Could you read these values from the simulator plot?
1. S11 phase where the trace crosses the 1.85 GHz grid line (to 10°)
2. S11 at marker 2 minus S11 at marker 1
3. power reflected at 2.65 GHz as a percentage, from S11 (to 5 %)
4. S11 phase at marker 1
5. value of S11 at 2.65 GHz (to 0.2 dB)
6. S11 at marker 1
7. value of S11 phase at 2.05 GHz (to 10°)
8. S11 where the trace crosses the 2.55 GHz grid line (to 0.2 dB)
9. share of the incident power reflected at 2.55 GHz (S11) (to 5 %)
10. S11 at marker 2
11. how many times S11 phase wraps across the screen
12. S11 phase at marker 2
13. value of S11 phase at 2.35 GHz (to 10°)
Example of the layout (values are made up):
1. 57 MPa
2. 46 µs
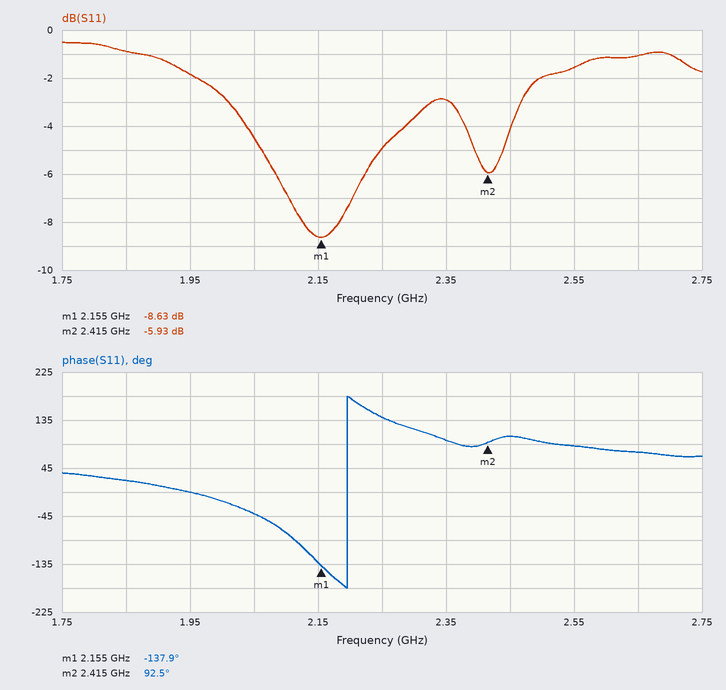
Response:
1. 20°
2. 2.70 dB
3. 80 %
4. -137.9°
5. -1.0 dB
6. -8.63 dB
7. -40°
8. -1.6 dB
9. 70 %
10. -5.93 dB
11. 1
12. 92.5°
13. 100°
